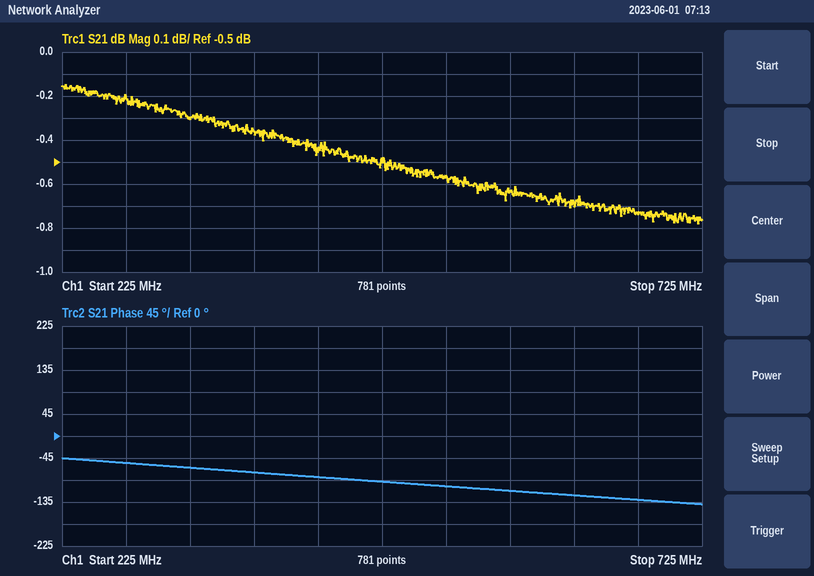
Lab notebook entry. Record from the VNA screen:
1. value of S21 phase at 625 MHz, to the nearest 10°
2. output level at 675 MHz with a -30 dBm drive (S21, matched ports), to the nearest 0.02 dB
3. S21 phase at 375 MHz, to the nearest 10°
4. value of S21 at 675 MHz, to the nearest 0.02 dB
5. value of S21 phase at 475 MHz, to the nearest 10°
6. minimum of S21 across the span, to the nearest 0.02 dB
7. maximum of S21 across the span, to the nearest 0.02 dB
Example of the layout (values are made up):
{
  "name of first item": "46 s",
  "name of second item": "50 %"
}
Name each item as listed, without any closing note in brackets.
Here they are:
{
  "value of S21 phase at 625 MHz, to the nearest 10°": "-120°",
  "output level at 675 MHz with a -30 dBm drive (S21, matched ports), to the nearest 0.02 dB": "-30.74 dBm",
  "S21 phase at 375 MHz, to the nearest 10°": "-70°",
  "value of S21 at 675 MHz, to the nearest 0.02 dB": "-0.74 dB",
  "value of S21 phase at 475 MHz, to the nearest 10°": "-90°",
  "minimum of S21 across the span, to the nearest 0.02 dB": "-0.78 dB",
  "maximum of S21 across the span, to the nearest 0.02 dB": "-0.14 dB"
}
